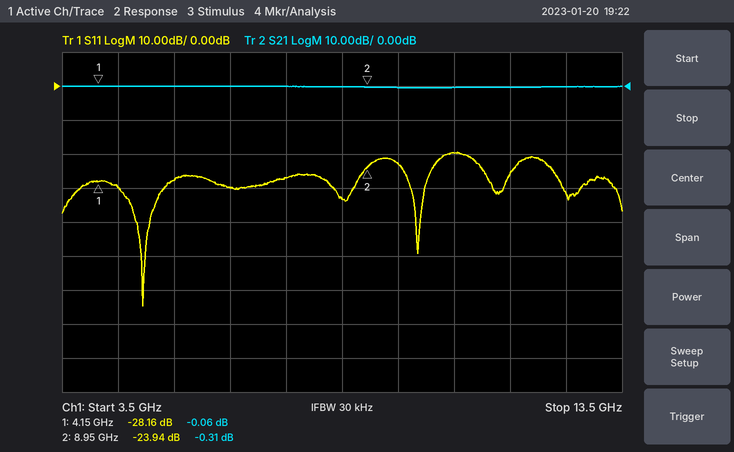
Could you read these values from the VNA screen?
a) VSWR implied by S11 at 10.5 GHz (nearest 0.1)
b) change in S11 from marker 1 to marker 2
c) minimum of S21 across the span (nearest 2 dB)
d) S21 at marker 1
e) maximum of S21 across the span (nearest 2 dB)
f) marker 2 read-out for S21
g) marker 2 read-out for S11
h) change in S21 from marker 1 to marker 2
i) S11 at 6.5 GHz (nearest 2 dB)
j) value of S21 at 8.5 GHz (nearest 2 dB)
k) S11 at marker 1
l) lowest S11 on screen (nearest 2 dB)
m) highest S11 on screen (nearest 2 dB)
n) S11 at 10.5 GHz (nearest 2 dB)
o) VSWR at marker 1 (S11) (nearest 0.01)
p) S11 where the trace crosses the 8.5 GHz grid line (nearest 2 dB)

1.2
4.22 dB
0 dB
-0.06 dB
0 dB
-0.31 dB
-23.94 dB
-0.25 dB
-30 dB
0 dB
-28.16 dB
-64 dB
-20 dB
-20 dB
1.08
-34 dB
